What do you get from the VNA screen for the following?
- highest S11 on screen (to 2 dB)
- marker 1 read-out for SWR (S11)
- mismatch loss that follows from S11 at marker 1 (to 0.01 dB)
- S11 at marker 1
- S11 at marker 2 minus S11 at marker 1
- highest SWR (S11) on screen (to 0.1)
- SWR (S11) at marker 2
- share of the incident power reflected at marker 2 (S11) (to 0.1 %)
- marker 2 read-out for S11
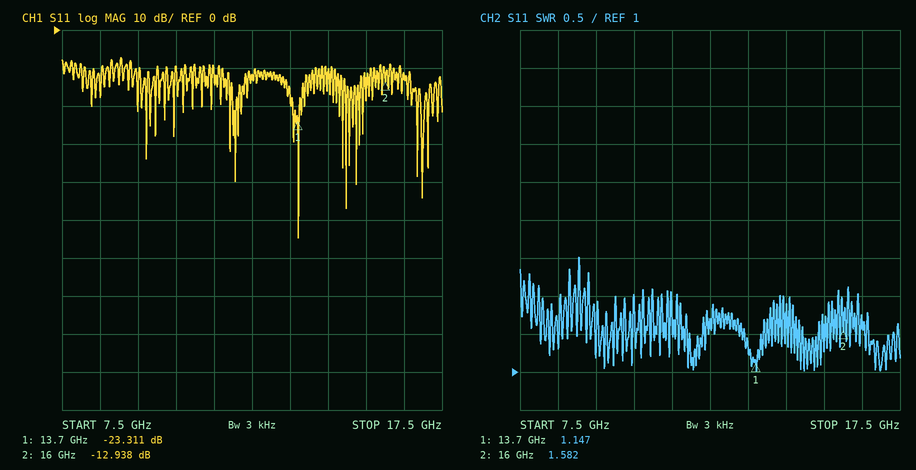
-8 dB
1.147
0.02 dB
-23.311 dB
10.373 dB
2.5
1.582
5.1 %
-12.938 dB
